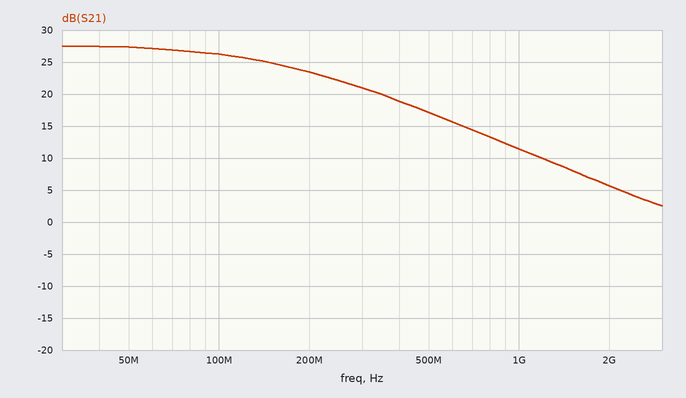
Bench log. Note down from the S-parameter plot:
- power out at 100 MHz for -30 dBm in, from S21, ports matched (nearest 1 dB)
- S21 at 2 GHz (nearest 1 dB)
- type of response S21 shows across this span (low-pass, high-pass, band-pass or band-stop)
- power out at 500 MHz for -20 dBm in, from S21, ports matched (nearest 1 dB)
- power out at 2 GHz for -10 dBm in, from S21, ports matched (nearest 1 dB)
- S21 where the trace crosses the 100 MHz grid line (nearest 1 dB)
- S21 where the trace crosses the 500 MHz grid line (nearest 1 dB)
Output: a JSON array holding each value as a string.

["-4 dBm", "6 dB", "low-pass", "-3 dBm", "-4 dBm", "26 dB", "17 dB"]
